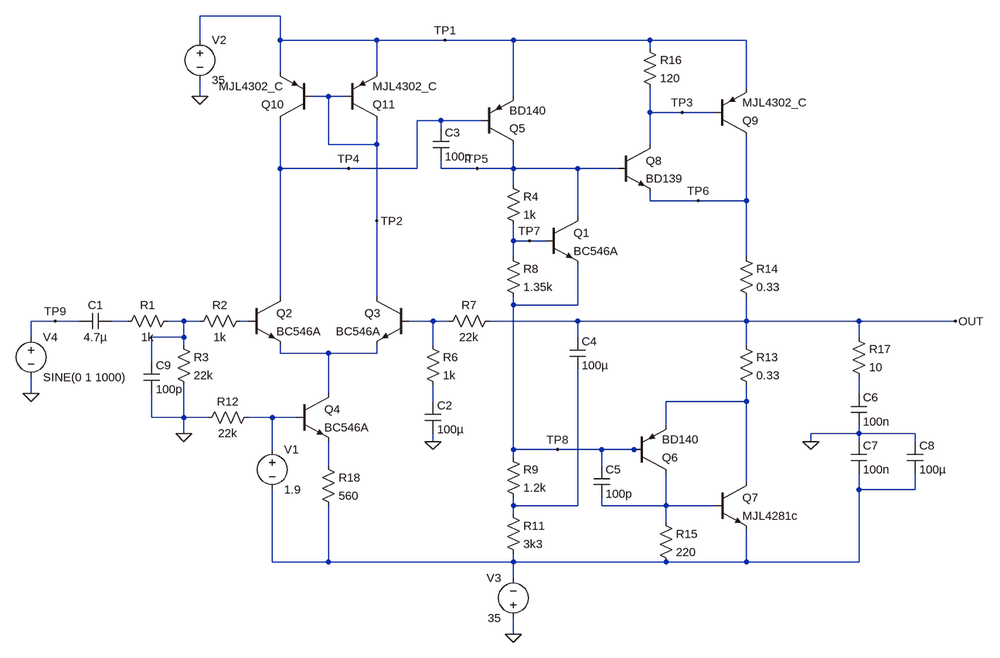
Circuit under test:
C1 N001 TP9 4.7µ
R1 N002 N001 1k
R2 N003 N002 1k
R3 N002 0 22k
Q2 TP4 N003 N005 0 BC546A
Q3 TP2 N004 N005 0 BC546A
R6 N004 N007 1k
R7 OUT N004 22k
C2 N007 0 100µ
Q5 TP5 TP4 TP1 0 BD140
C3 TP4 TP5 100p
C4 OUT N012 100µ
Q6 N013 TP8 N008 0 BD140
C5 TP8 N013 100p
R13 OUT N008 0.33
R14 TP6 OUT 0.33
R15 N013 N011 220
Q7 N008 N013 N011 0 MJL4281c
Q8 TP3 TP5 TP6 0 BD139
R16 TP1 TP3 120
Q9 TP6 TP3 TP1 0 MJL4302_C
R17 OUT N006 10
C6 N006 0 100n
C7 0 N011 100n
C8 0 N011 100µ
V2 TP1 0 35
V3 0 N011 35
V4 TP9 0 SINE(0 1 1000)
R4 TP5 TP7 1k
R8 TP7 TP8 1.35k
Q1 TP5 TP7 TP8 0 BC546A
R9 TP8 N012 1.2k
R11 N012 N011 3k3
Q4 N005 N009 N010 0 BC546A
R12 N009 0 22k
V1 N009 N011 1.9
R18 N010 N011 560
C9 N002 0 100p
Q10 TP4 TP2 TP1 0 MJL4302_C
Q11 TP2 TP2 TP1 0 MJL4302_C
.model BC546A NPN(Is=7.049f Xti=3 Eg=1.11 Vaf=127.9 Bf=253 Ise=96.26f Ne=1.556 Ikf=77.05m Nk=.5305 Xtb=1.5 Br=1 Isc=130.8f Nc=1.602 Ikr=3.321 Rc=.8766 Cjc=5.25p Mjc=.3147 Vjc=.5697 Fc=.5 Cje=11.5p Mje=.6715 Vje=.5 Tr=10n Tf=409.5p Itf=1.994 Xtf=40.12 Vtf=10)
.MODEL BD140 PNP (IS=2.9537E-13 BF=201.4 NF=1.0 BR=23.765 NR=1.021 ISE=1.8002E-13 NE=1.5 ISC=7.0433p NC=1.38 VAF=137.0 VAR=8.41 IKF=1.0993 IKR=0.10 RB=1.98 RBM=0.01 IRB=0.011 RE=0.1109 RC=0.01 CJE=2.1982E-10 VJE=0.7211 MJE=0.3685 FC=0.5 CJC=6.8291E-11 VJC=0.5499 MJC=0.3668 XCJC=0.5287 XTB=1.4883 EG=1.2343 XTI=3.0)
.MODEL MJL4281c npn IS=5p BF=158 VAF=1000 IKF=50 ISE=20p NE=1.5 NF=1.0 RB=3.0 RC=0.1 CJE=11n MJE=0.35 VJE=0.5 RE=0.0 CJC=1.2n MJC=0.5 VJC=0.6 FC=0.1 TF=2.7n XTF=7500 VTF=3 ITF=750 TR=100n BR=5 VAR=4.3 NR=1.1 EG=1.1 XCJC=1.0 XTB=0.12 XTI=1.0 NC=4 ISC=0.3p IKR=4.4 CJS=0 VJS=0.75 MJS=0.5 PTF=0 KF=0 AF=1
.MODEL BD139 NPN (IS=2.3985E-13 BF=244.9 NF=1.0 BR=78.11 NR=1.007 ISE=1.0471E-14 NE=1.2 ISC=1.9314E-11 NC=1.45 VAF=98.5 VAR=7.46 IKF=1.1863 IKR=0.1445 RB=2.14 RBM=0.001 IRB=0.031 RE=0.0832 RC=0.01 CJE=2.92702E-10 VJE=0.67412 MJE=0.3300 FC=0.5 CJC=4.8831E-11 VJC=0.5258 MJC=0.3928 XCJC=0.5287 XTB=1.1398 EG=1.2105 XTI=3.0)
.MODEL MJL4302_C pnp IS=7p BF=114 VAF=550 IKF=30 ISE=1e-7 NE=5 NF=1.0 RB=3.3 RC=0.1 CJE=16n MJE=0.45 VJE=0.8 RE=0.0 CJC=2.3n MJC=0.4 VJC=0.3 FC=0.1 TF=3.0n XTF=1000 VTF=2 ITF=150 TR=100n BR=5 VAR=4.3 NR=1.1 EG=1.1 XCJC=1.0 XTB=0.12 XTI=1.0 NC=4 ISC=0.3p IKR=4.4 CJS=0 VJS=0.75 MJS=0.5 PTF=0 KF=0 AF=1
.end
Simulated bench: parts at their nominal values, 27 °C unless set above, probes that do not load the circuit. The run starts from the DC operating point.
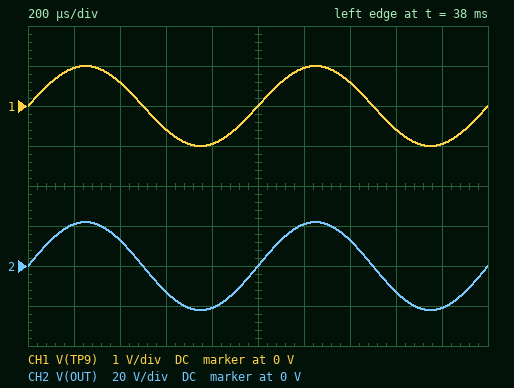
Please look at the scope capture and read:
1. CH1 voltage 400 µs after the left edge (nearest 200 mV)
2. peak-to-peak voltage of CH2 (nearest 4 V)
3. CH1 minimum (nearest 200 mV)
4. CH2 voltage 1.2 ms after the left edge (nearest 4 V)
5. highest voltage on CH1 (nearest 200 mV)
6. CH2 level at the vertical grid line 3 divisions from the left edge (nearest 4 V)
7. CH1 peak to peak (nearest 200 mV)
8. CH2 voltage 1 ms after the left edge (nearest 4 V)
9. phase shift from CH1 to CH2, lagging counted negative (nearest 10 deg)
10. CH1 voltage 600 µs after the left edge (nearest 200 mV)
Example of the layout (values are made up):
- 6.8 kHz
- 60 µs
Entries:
- 600 mV
- 44 V
- -1.0 V
- 20 V
- 1.0 V
- -12 V
- 2.0 V
- 0 V
- 0 deg
- -600 mV
